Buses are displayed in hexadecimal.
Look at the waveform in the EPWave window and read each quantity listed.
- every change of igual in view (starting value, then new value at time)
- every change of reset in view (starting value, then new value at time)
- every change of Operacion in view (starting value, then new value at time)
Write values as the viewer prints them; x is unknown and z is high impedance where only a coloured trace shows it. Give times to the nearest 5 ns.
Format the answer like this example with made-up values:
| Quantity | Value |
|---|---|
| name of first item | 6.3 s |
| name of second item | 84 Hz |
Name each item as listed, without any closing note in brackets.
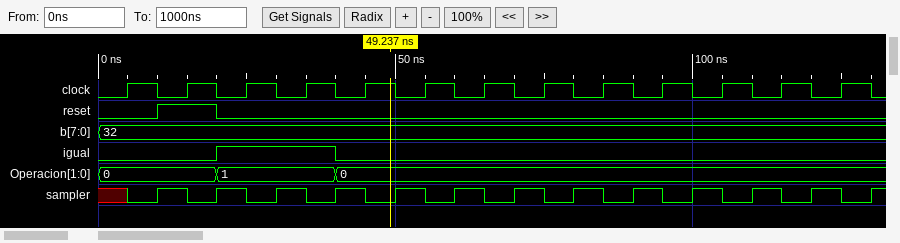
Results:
| Quantity | Value |
|---|---|
| every change of igual in view | 0, 1 at 20 ns, 0 at 40 ns |
| every change of reset in view | 0, 1 at 10 ns, 0 at 20 ns |
| every change of Operacion in view | 0, 1 at 20 ns, 0 at 40 ns |
